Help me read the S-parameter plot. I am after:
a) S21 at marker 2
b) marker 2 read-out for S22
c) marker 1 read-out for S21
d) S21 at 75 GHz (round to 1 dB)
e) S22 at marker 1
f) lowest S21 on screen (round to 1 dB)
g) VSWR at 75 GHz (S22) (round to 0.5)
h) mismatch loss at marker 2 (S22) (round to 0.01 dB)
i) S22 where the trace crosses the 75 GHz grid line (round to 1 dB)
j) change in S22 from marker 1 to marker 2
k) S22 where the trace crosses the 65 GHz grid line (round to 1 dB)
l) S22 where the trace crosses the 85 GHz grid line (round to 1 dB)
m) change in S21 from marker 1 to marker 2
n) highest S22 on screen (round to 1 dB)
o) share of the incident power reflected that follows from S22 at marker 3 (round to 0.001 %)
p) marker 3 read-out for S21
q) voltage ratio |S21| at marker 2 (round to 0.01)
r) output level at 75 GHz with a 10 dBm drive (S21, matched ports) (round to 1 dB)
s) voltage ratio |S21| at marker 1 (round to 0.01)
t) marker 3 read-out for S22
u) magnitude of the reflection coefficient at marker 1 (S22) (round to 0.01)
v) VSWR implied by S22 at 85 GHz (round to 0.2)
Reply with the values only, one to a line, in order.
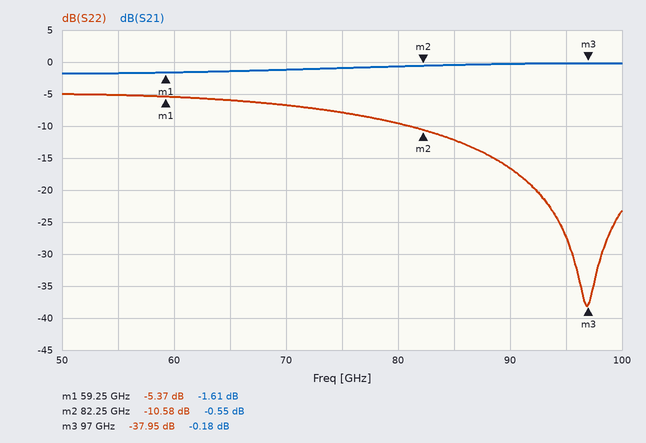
-0.55 dB
-10.58 dB
-1.61 dB
-1 dB
-5.37 dB
-2 dB
2.5
0.40 dB
-8 dB
-5.21 dB
-6 dB
-12 dB
1.06 dB
-5 dB
0.016 %
-0.18 dB
0.94
9 dBm
0.83
-37.95 dB
0.54
1.6
